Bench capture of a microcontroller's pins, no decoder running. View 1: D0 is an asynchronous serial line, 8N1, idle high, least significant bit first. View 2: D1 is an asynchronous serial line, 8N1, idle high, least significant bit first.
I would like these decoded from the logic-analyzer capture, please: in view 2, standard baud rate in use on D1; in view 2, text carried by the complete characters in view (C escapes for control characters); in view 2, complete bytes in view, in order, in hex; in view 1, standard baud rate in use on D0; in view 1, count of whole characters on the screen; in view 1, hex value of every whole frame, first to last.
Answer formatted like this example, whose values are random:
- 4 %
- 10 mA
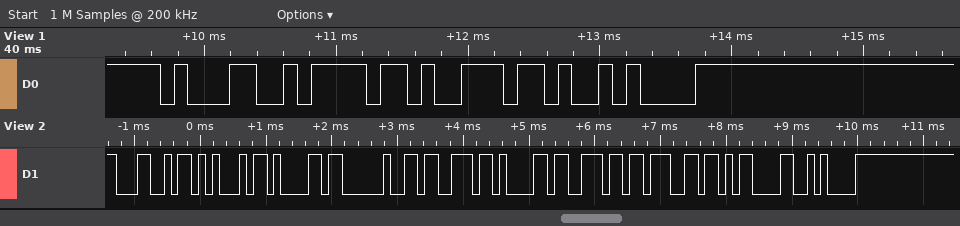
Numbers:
- 9600 baud
- "LEa sang\r\n"
- 4C 45 61 20 73 61 6E 67 0D 0A
- 9600 baud
- 4
- 0x31 0x6F 0x6E 0x0A
